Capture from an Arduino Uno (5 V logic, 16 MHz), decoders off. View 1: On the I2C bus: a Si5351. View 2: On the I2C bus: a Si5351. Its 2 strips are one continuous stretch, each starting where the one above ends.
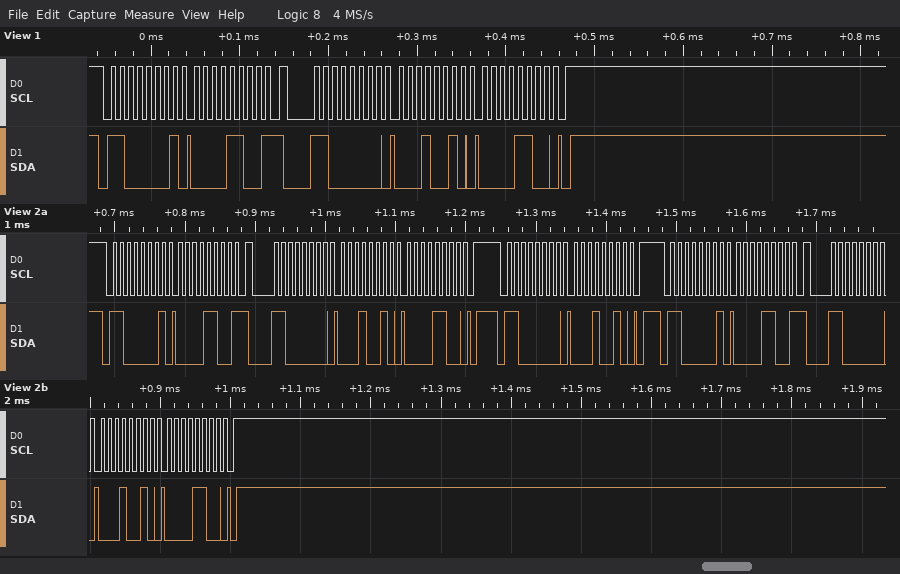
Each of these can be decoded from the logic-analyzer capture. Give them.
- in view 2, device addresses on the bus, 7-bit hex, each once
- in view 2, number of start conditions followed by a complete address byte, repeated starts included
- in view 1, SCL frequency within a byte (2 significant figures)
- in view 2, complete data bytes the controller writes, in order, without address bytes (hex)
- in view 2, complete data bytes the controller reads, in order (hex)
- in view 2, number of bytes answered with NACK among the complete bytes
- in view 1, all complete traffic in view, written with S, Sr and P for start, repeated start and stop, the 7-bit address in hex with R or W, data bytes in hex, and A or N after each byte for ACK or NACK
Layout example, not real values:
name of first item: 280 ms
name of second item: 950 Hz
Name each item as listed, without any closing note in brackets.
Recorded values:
in view 2, device addresses on the bus, 7-bit hex, each once: 0x60
in view 2, number of start conditions followed by a complete address byte, repeated starts included: 5
in view 1, SCL frequency within a byte: 100 kHz
in view 2, complete data bytes the controller writes, in order, without address bytes: 12 0C 12 12 0C
in view 2, complete data bytes the controller reads, in order: 0C 0C
in view 2, number of bytes answered with NACK among the complete bytes: 2
in view 1, all complete traffic in view, written with S, Sr and P for start, repeated start and stop, the 7-bit address in hex with R or W, data bytes in hex, and A or N after each byte for ACK or NACK: S 60R A 0C N Sr 60W A 12 A 0C A P
